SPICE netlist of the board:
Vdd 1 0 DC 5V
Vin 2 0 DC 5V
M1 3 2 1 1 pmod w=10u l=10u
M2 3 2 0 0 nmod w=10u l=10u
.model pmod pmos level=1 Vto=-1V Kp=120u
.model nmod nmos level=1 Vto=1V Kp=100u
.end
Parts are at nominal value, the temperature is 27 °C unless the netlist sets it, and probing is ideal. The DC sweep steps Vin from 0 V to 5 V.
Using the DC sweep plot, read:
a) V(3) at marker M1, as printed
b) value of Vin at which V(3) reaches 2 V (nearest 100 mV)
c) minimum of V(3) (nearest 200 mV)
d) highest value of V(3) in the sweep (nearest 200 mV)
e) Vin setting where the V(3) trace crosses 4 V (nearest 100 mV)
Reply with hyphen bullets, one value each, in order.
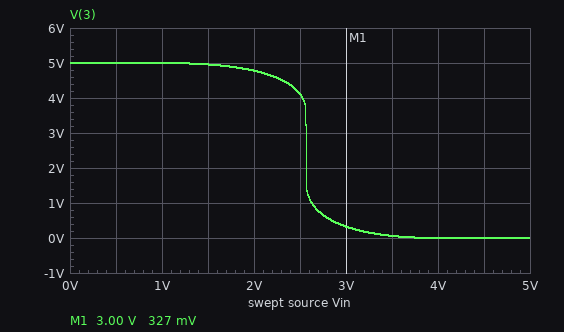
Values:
- 327 mV
- 2.6 V
- 0 V
- 5.0 V
- 2.5 V
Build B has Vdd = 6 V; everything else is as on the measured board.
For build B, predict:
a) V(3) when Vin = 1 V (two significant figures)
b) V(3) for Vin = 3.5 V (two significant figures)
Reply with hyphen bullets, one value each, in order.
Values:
- 6.0 V
- 620 mV
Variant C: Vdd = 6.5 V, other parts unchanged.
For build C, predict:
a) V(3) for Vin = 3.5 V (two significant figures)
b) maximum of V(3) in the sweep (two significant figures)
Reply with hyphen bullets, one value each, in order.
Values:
- 1.3 V
- 6.5 V
